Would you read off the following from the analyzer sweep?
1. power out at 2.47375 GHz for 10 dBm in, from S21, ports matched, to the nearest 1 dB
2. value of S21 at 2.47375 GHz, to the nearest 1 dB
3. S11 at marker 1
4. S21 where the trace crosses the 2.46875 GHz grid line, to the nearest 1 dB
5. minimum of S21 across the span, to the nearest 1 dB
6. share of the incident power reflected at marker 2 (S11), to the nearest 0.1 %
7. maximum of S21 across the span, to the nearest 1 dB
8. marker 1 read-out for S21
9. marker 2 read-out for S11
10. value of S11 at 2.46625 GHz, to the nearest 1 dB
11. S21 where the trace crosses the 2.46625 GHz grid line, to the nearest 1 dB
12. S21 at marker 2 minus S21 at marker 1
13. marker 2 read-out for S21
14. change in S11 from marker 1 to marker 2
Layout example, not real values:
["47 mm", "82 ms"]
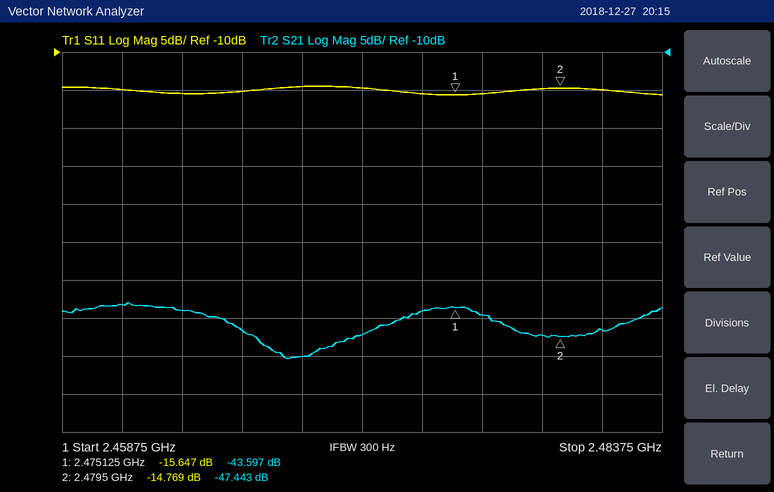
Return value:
["-34 dBm", "-44 dB", "-15.647 dB", "-50 dB", "-50 dB", "3.3 %", "-43 dB", "-43.597 dB", "-14.769 dB", "-15 dB", "-47 dB", "-3.846 dB", "-47.443 dB", "0.878 dB"]
